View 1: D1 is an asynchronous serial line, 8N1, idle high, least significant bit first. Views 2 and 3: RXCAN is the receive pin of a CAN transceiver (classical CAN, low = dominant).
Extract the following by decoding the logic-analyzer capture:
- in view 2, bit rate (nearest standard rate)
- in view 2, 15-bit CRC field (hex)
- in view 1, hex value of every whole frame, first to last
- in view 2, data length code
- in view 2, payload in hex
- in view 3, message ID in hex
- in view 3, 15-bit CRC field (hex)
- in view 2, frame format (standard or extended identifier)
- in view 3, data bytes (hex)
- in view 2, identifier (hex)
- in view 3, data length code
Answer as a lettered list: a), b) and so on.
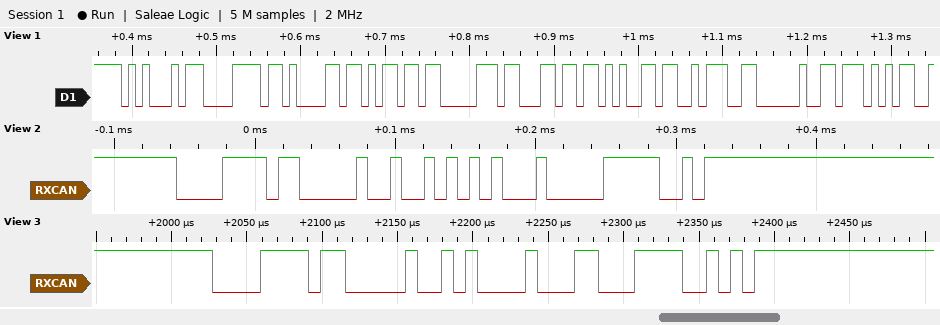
a) 125 kbit/s
b) 0x441E
c) 45 78 61 6D 70 6C 65 3A 20 57
d) 1
e) 2A
f) 0x0F6
g) 0x18F2
h) standard
i) 42
j) 0x0F6
k) 1
